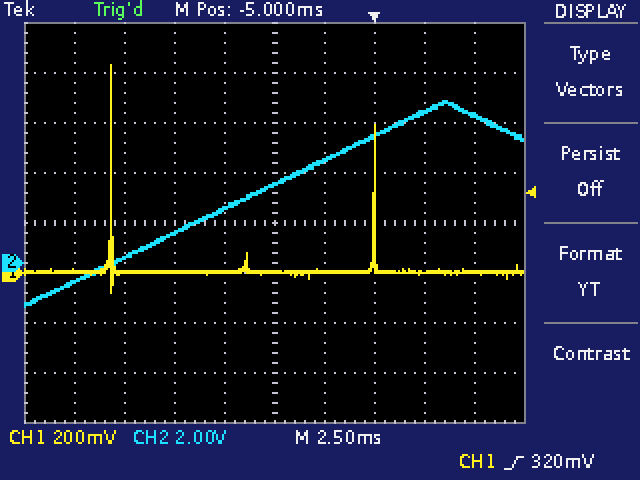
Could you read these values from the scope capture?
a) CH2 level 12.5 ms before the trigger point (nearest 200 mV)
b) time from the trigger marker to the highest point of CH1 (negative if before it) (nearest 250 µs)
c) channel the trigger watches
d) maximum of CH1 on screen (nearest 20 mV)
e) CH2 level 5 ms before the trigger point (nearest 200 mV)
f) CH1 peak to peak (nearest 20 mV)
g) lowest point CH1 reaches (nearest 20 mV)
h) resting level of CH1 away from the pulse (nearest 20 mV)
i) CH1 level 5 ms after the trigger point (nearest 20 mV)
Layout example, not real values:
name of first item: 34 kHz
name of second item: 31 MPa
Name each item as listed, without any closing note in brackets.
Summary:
CH2 level 12.5 ms before the trigger point: 200 mV
time from the trigger marker to the highest point of CH1 (negative if before it): -13.25 ms
channel the trigger watches: CH1
maximum of CH1 on screen: 840 mV
CH2 level 5 ms before the trigger point: 3.2 V
CH1 peak to peak: 920 mV
lowest point CH1 reaches: -80 mV
resting level of CH1 away from the pulse: 0 mV
CH1 level 5 ms after the trigger point: 0 mV
